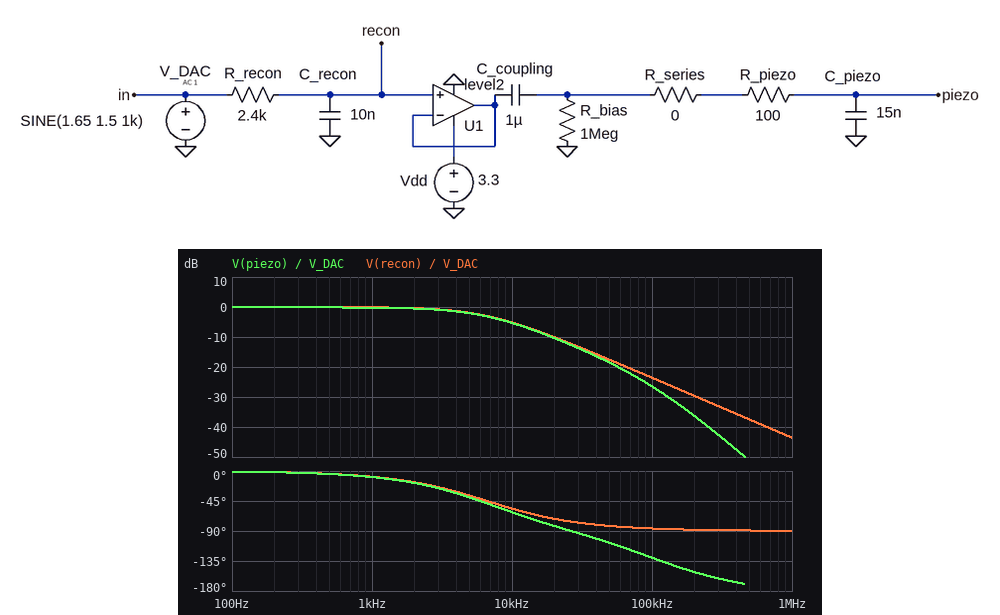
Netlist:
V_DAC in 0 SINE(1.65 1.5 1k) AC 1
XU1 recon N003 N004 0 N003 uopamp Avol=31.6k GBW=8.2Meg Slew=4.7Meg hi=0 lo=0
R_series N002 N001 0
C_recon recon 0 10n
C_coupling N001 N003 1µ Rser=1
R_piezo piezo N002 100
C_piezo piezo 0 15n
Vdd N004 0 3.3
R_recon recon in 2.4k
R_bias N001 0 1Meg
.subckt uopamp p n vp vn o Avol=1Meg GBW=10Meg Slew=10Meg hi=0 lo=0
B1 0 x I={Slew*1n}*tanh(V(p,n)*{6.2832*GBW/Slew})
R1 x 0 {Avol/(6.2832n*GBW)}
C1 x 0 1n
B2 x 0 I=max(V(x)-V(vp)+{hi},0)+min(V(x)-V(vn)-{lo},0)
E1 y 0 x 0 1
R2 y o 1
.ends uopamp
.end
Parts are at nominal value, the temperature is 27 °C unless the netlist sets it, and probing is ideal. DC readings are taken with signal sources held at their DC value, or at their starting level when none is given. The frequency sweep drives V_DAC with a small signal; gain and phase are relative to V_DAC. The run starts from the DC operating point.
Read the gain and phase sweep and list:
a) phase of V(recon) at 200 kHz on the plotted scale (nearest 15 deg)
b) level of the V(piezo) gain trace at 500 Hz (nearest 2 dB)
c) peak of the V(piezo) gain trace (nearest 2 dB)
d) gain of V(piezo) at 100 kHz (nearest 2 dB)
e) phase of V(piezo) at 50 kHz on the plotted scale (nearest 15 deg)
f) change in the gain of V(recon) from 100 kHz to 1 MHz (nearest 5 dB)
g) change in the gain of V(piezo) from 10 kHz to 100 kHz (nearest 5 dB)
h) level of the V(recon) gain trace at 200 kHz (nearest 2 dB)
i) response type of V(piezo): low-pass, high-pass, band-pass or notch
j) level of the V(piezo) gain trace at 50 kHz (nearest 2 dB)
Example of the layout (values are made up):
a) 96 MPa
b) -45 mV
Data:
a) -90 deg
b) 0 dB
c) 0 dB
d) -26 dB
e) -105 deg
f) -20 dB
g) -20 dB
h) -30 dB
i) low-pass
j) -18 dB
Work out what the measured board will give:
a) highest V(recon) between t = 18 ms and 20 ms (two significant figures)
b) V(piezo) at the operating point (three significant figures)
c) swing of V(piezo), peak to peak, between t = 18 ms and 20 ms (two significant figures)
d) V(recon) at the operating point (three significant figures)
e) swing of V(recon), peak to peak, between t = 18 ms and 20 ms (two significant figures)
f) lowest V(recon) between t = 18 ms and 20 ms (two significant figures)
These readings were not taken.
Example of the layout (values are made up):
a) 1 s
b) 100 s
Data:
a) 3.1 V
b) 1.62 V
c) 2.9 V
d) 1.65 V
e) 3.0 V
f) 170 mV
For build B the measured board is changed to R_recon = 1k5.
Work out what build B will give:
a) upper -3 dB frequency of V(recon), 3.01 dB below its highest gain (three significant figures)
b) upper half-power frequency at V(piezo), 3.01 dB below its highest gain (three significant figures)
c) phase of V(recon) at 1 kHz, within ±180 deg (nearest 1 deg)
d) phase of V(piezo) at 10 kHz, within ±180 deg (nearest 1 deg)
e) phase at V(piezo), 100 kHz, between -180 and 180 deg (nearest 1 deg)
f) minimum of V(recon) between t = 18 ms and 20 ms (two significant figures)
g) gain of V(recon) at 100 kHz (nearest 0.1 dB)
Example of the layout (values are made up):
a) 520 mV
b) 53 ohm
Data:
a) 10.6 kHz
b) 10.5 kHz
c) -5 deg
d) -49 deg
e) -128 deg
f) 160 mV
g) -19.5 dB
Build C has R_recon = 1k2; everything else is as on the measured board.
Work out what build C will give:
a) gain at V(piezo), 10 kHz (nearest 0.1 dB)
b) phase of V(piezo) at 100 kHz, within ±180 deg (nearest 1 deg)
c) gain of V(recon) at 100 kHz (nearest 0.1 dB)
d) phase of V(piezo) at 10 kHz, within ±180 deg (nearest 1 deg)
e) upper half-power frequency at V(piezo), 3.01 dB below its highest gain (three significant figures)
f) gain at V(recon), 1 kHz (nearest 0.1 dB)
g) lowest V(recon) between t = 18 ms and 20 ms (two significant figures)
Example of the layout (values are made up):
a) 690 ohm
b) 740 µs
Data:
a) -2.1 dB
b) -126 deg
c) -17.6 dB
d) -42 deg
e) 13.1 kHz
f) 0 dB
g) 150 mV
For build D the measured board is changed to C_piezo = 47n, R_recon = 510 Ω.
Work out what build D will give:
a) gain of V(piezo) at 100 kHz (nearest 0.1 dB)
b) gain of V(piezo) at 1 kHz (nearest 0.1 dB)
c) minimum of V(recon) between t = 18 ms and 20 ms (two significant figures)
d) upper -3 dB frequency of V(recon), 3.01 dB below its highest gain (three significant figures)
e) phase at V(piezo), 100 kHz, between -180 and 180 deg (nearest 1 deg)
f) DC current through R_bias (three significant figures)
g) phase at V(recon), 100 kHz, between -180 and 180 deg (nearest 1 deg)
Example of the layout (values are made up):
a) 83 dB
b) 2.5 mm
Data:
a) -20.5 dB
b) -0.4 dB
c) 150 mV
d) 31.2 kHz
e) -144 deg
f) 1.58 µA
g) -73 deg
